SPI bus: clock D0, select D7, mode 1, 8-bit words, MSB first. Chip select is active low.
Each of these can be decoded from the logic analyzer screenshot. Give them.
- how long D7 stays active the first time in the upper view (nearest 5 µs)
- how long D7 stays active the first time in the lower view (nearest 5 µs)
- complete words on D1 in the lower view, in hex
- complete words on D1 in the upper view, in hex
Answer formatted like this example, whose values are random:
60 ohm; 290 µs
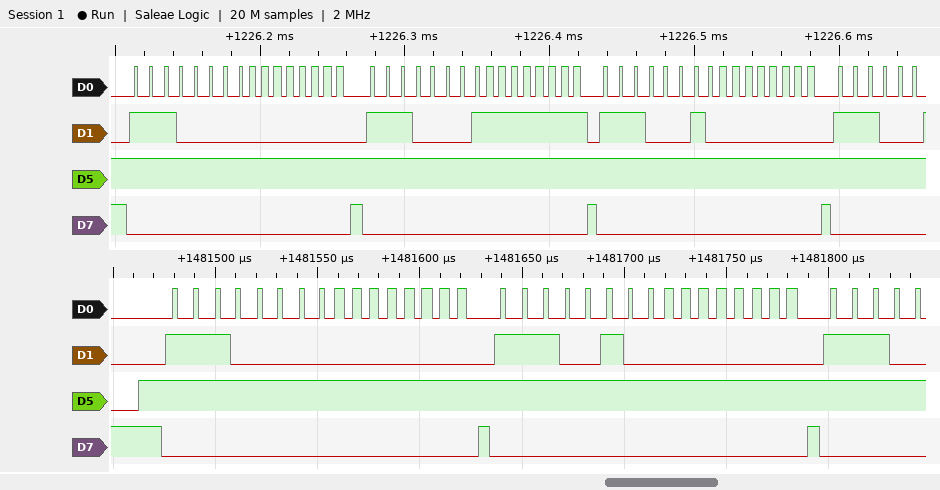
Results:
155 µs; 155 µs; E0, 00, E4, 00; E0, 00, E1, FF, E2, 00
